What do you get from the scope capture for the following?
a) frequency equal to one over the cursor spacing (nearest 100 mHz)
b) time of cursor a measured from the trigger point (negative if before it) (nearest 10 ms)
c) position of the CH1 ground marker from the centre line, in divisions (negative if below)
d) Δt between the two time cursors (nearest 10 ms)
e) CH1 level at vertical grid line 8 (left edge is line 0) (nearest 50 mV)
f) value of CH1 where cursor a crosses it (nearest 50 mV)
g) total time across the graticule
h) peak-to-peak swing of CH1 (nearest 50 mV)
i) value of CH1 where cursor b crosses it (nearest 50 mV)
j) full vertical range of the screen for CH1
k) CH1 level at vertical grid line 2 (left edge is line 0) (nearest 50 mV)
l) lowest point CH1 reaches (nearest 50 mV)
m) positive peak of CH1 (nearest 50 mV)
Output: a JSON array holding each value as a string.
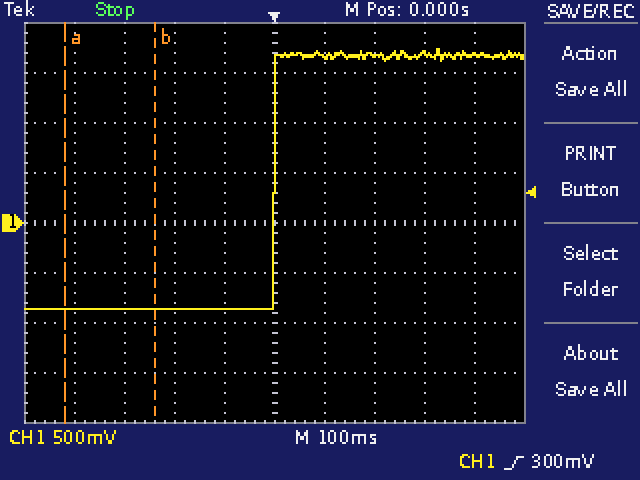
["5.6 Hz", "-420 ms", "0.0 div", "180 ms", "1.70 V", "-850 mV", "1 s", "2.60 V", "-850 mV", "4 V", "-850 mV", "-850 mV", "1.75 V"]
